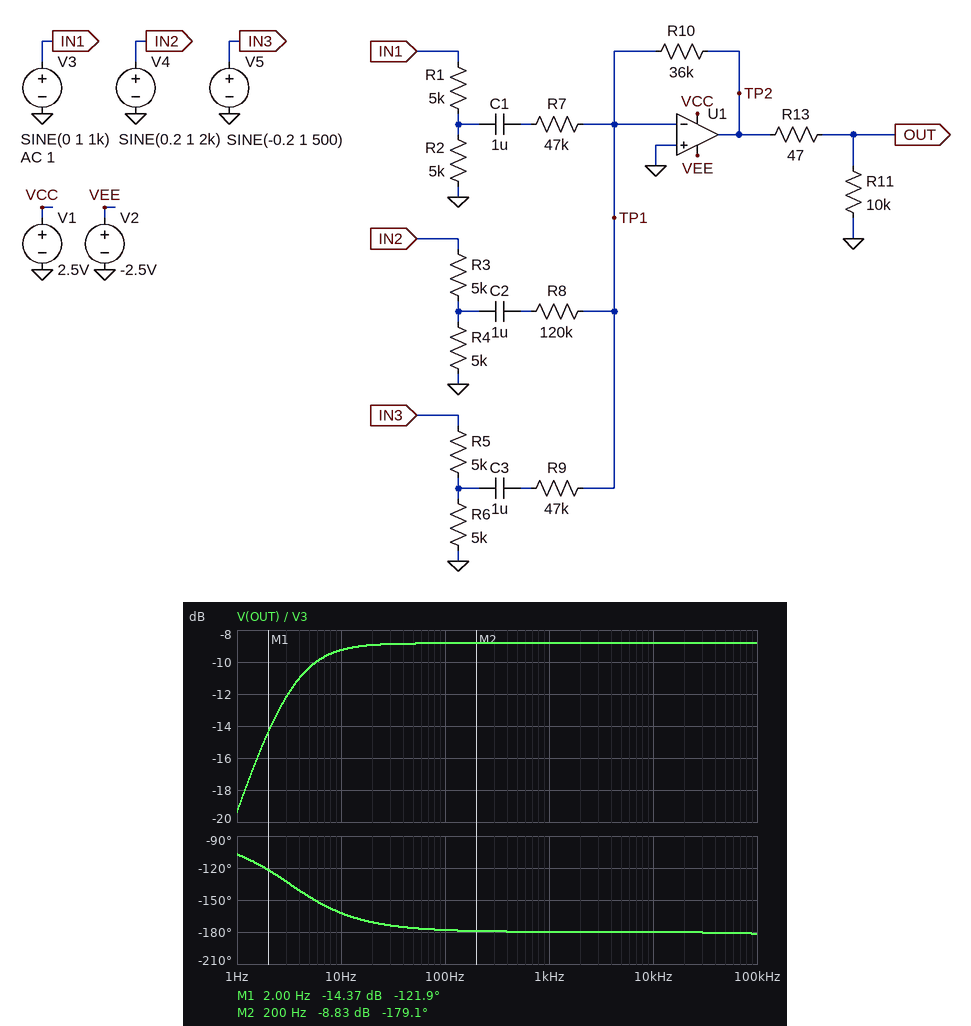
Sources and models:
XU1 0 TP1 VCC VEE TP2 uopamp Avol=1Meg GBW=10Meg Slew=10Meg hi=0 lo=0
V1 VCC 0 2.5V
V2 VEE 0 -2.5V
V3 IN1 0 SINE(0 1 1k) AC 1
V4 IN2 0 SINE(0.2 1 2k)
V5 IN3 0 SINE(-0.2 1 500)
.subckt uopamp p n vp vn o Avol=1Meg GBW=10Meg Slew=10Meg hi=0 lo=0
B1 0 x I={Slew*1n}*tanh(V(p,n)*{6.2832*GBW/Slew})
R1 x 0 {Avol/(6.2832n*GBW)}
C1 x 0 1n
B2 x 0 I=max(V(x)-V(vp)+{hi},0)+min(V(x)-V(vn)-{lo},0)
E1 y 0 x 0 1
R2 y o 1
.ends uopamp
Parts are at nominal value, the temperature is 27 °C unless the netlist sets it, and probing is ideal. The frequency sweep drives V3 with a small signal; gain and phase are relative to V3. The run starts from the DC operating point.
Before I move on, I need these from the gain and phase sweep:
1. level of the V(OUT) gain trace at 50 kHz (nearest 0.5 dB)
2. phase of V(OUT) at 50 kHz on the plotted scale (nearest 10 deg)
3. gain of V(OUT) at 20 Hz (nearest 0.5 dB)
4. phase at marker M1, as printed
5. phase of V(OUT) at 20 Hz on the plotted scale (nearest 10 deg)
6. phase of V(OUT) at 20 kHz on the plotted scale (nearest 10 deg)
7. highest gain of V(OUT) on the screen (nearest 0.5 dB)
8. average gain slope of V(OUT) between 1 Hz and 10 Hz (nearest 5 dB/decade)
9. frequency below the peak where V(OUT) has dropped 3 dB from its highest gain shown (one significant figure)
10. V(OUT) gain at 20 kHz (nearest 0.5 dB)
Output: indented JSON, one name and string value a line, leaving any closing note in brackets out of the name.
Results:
{
  "level of the V(OUT) gain trace at 50 kHz": "-9.0 dB",
  "phase of V(OUT) at 50 kHz on the plotted scale": "-180 deg",
  "gain of V(OUT) at 20 Hz": "-9.0 dB",
  "phase at marker M1, as printed": "-121.9 deg",
  "phase of V(OUT) at 20 Hz on the plotted scale": "-170 deg",
  "phase of V(OUT) at 20 kHz on the plotted scale": "-180 deg",
  "highest gain of V(OUT) on the screen": "-9.0 dB",
  "average gain slope of V(OUT) between 1 Hz and 10 Hz": "10 dB/decade",
  "frequency below the peak where V(OUT) has dropped 3 dB from its highest gain shown": "3 Hz",
  "V(OUT) gain at 20 kHz": "-9.0 dB"
}
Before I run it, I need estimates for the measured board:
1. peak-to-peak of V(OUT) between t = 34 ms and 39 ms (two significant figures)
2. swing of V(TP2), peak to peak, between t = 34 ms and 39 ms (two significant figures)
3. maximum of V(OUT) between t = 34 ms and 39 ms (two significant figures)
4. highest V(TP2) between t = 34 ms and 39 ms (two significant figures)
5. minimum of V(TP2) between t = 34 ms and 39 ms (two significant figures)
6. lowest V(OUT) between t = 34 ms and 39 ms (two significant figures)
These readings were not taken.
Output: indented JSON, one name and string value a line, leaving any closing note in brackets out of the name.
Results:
{
  "peak-to-peak of V(OUT) between t = 34 ms and 39 ms": "1.3 V",
  "swing of V(TP2), peak to peak, between t = 34 ms and 39 ms": "1.3 V",
  "maximum of V(OUT) between t = 34 ms and 39 ms": "640 mV",
  "highest V(TP2) between t = 34 ms and 39 ms": "650 mV",
  "minimum of V(TP2) between t = 34 ms and 39 ms": "-650 mV",
  "lowest V(OUT) between t = 34 ms and 39 ms": "-640 mV"
}
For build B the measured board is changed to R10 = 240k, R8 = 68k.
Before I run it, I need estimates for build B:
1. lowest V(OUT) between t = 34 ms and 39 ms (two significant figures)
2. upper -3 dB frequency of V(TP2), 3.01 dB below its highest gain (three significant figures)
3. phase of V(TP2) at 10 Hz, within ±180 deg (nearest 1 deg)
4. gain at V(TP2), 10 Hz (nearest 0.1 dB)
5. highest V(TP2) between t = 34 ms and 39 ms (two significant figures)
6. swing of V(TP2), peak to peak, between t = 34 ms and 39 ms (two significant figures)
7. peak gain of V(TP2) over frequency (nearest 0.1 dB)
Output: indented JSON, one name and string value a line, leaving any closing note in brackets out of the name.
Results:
{
  "lowest V(OUT) between t = 34 ms and 39 ms": "-2.5 V",
  "upper -3 dB frequency of V(TP2), 3.01 dB below its highest gain": "709 kHz",
  "phase of V(TP2) at 10 Hz, within ±180 deg": "-162 deg",
  "gain at V(TP2), 10 Hz": "7.3 dB",
  "highest V(TP2) between t = 34 ms and 39 ms": "2.5 V",
  "swing of V(TP2), peak to peak, between t = 34 ms and 39 ms": "5.0 V",
  "peak gain of V(TP2) over frequency": "7.7 dB"
}
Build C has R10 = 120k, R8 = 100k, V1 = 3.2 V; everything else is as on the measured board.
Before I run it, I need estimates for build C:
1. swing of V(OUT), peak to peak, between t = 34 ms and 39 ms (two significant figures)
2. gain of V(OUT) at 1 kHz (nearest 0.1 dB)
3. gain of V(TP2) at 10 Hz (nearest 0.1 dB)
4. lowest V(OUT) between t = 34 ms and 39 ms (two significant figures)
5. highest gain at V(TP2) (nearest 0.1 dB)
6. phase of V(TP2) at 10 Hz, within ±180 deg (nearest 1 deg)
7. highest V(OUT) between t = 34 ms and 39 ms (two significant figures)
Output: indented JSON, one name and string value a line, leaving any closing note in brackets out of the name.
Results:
{
  "swing of V(OUT), peak to peak, between t = 34 ms and 39 ms": "4.4 V",
  "gain of V(OUT) at 1 kHz": "1.6 dB",
  "gain of V(TP2) at 10 Hz": "1.2 dB",
  "lowest V(OUT) between t = 34 ms and 39 ms": "-2.2 V",
  "highest gain at V(TP2)": "1.7 dB",
  "phase of V(TP2) at 10 Hz, within ±180 deg": "-162 deg",
  "highest V(OUT) between t = 34 ms and 39 ms": "2.2 V"
}
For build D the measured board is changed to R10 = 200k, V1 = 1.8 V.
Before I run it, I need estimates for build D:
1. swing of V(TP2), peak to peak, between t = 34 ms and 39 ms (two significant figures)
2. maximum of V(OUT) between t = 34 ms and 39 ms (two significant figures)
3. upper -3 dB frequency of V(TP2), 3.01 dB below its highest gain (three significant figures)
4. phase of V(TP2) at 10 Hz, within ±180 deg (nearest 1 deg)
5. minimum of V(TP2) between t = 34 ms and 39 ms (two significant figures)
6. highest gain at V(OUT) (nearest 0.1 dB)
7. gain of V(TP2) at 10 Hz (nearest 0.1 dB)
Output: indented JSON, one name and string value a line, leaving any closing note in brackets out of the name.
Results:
{
  "swing of V(TP2), peak to peak, between t = 34 ms and 39 ms": "4.3 V",
  "maximum of V(OUT) between t = 34 ms and 39 ms": "1.8 V",
  "upper -3 dB frequency of V(TP2), 3.01 dB below its highest gain": "933 kHz",
  "phase of V(TP2) at 10 Hz, within ±180 deg": "-162 deg",
  "minimum of V(TP2) between t = 34 ms and 39 ms": "-2.5 V",
  "highest gain at V(OUT)": "6.1 dB",
  "gain of V(TP2) at 10 Hz": "5.7 dB"
}
